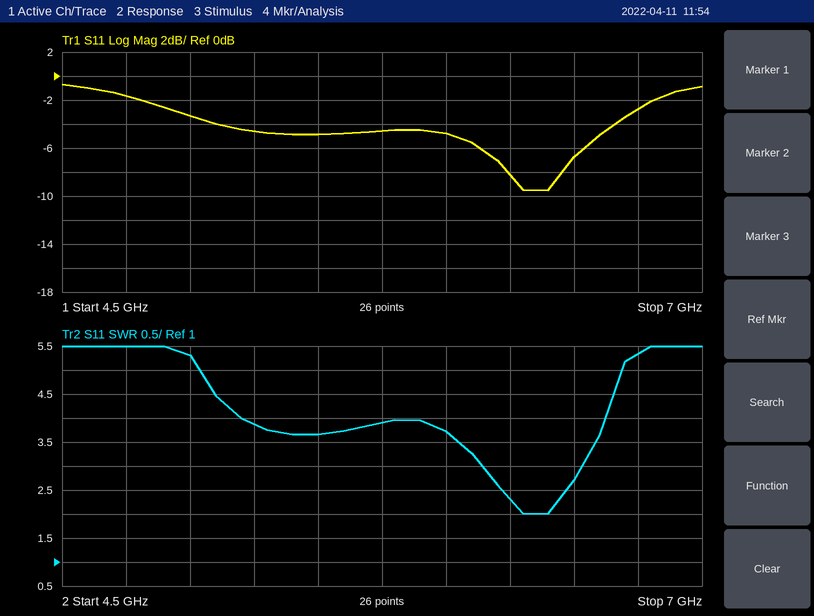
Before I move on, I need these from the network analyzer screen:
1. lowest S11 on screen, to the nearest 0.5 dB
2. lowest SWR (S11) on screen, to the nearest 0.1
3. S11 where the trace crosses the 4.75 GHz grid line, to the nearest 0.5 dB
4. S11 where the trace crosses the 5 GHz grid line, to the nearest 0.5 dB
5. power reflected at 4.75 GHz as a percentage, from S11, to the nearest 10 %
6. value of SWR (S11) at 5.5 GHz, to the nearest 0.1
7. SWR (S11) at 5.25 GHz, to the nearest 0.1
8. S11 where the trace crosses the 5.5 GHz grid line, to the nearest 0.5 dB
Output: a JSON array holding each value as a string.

["-9.5 dB", "2.0", "-1.5 dB", "-3.5 dB", "70 %", "3.7", "3.9", "-5.0 dB"]
